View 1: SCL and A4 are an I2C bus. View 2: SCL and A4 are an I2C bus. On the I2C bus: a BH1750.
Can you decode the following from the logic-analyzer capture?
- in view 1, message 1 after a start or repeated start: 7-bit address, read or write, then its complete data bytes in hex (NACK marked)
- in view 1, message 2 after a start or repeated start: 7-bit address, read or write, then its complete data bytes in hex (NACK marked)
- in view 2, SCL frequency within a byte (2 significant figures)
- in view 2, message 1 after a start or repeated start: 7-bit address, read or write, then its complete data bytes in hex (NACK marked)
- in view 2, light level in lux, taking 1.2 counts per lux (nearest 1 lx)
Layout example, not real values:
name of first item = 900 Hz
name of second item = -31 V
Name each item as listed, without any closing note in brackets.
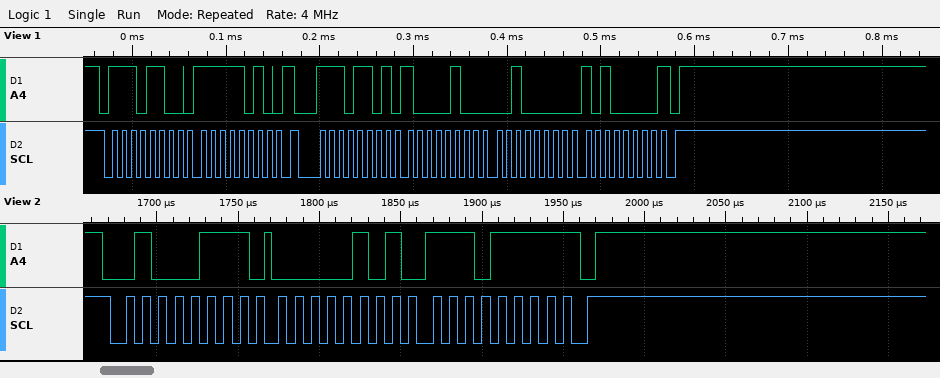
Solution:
in view 1, message 1 after a start or repeated start: 7-bit address, read or write, then its complete data bytes in hex = 0x76 write: FA
in view 1, message 2 after a start or repeated start: 7-bit address, read or write, then its complete data bytes in hex = 0x76 read: 84 20 A0 NACK
in view 2, SCL frequency within a byte = 100 kHz
in view 2, message 1 after a start or repeated start: 7-bit address, read or write, then its complete data bytes in hex = 0x23 read: 05 EF NACK
in view 2, light level in lux, taking 1.2 counts per lux = 1266 lx
